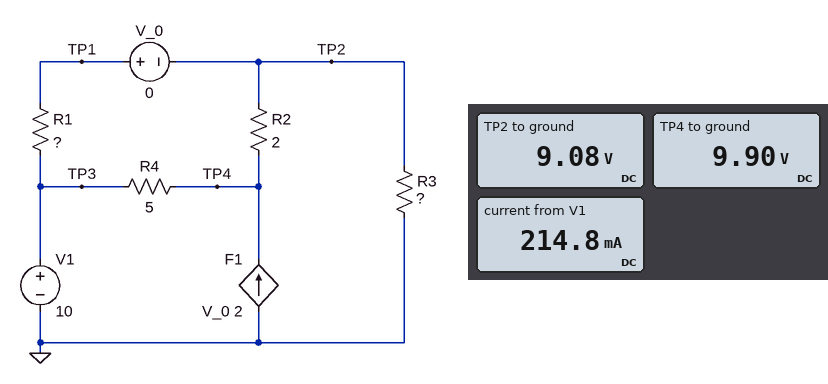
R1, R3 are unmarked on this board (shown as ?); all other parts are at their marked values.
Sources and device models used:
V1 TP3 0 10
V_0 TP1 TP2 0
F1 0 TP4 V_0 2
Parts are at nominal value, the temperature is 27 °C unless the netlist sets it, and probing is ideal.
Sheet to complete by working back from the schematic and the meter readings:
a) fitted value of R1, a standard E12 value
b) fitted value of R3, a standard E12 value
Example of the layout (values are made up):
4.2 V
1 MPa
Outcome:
4.7 Ω
15 Ω
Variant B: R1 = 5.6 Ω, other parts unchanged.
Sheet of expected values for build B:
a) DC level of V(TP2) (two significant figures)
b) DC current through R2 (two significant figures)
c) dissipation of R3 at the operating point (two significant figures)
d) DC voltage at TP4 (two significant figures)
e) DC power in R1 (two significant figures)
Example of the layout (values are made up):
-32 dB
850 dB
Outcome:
9.0 V
410 mA
5.4 W
9.8 V
190 mW
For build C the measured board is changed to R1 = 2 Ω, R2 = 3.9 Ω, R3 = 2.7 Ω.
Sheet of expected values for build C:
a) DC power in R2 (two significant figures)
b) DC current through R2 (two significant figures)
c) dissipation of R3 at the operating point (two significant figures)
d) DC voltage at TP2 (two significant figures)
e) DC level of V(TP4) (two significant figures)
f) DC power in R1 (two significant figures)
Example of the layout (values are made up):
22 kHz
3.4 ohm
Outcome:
10 W
1.6 A
21 W
7.6 V
14 V
2.9 W
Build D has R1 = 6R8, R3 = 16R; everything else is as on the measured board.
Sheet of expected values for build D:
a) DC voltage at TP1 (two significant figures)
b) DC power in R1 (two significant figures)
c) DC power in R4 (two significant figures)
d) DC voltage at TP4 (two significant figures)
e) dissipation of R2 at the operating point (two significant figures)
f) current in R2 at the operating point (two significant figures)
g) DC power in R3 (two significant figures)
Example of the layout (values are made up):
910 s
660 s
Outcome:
8.9 V
180 mW
21 mW
9.7 V
310 mW
390 mA
4.9 W
